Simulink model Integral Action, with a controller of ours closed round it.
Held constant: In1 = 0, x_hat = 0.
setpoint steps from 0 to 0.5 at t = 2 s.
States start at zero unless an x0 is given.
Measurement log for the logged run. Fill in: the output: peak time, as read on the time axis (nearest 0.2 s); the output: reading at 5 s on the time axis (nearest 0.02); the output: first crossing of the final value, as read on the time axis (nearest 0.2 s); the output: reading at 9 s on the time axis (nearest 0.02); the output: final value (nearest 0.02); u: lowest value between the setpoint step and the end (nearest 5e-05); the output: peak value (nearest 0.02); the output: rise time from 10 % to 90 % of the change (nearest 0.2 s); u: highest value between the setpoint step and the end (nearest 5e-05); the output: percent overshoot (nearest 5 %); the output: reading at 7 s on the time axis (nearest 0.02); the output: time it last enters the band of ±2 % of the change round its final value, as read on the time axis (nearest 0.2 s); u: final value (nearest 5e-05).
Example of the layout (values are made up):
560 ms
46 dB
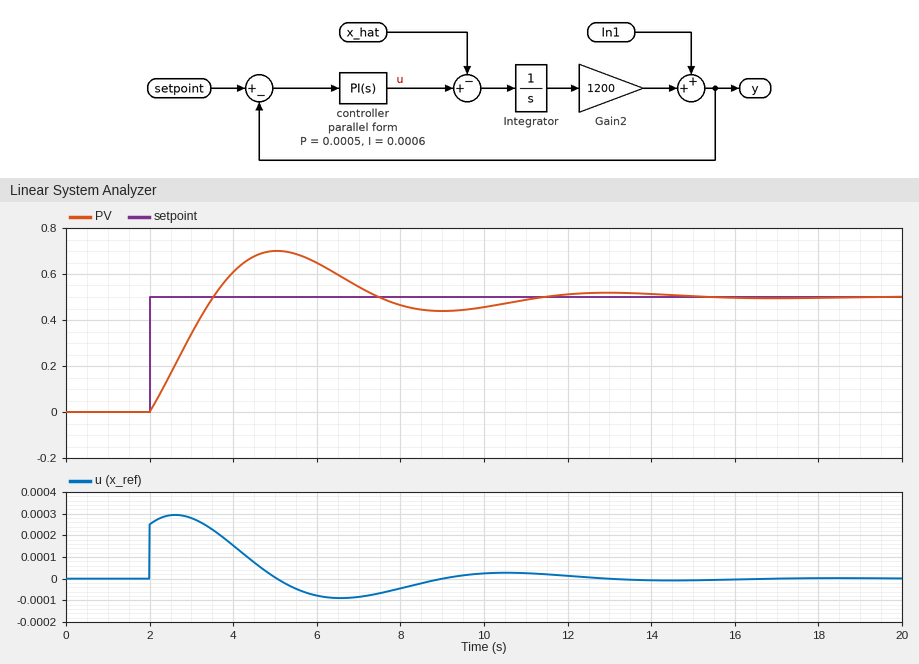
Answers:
5.0 s
0.70
3.6 s
0.44
0.50
-0.00010
0.70
1.2 s
0.00030
40 %
0.54
14.4 s
0.00000
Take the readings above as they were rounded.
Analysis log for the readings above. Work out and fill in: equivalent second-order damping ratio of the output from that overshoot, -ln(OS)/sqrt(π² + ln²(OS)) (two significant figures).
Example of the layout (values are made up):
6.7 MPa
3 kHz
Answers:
0.28
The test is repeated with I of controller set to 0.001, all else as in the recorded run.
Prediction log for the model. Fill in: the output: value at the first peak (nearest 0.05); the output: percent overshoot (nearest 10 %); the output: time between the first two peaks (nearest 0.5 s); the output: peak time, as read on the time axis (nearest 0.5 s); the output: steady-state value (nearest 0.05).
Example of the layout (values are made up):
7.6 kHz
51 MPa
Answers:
0.75
50 %
6.0 s
4.5 s
0.50
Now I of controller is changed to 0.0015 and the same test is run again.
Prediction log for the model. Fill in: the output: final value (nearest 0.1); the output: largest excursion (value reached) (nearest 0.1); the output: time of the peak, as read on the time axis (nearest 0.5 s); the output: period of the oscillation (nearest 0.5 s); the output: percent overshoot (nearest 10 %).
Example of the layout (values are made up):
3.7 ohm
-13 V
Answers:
0.5
0.8
4.0 s
5.0 s
50 %
